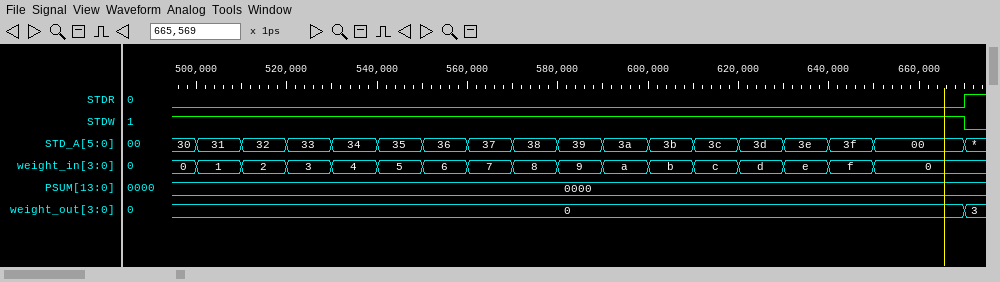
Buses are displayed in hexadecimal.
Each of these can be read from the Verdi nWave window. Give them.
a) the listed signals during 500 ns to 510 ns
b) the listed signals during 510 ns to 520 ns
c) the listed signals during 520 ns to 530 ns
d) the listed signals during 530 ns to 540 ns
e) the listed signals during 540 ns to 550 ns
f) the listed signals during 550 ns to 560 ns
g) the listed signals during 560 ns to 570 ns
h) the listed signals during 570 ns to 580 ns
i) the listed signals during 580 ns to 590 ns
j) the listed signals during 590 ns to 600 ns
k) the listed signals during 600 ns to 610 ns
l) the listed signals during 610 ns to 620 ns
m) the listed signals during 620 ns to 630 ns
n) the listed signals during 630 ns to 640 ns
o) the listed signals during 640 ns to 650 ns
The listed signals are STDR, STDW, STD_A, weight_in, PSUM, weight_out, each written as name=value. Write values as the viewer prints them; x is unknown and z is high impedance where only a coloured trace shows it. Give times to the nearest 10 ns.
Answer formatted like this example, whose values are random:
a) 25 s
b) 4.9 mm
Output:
a) STDR=0, STDW=1, STD_A=31, weight_in=1, PSUM=0000, weight_out=0
b) STDR=0, STDW=1, STD_A=32, weight_in=2, PSUM=0000, weight_out=0
c) STDR=0, STDW=1, STD_A=33, weight_in=3, PSUM=0000, weight_out=0
d) STDR=0, STDW=1, STD_A=34, weight_in=4, PSUM=0000, weight_out=0
e) STDR=0, STDW=1, STD_A=35, weight_in=5, PSUM=0000, weight_out=0
f) STDR=0, STDW=1, STD_A=36, weight_in=6, PSUM=0000, weight_out=0
g) STDR=0, STDW=1, STD_A=37, weight_in=7, PSUM=0000, weight_out=0
h) STDR=0, STDW=1, STD_A=38, weight_in=8, PSUM=0000, weight_out=0
i) STDR=0, STDW=1, STD_A=39, weight_in=9, PSUM=0000, weight_out=0
j) STDR=0, STDW=1, STD_A=3a, weight_in=a, PSUM=0000, weight_out=0
k) STDR=0, STDW=1, STD_A=3b, weight_in=b, PSUM=0000, weight_out=0
l) STDR=0, STDW=1, STD_A=3c, weight_in=c, PSUM=0000, weight_out=0
m) STDR=0, STDW=1, STD_A=3d, weight_in=d, PSUM=0000, weight_out=0
n) STDR=0, STDW=1, STD_A=3e, weight_in=e, PSUM=0000, weight_out=0
o) STDR=0, STDW=1, STD_A=3f, weight_in=f, PSUM=0000, weight_out=0
